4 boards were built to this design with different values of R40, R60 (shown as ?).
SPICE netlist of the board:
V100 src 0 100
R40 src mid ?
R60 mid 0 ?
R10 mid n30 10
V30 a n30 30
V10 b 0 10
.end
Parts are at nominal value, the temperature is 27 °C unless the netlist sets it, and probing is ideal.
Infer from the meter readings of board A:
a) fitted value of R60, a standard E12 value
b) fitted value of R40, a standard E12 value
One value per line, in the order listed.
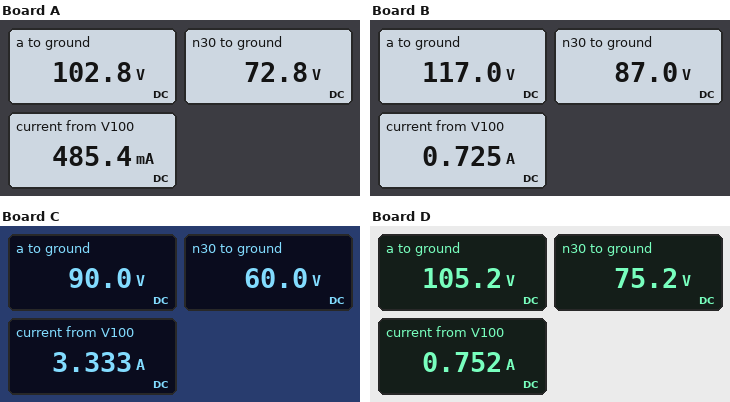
150 Ω
56 Ω
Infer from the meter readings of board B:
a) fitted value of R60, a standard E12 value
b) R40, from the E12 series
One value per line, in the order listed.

120 Ω
18 Ω
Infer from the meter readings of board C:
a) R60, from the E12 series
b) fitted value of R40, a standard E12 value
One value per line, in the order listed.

18 Ω
12 Ω
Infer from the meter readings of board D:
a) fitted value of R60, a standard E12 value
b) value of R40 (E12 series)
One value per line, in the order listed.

100 Ω
33 Ω
